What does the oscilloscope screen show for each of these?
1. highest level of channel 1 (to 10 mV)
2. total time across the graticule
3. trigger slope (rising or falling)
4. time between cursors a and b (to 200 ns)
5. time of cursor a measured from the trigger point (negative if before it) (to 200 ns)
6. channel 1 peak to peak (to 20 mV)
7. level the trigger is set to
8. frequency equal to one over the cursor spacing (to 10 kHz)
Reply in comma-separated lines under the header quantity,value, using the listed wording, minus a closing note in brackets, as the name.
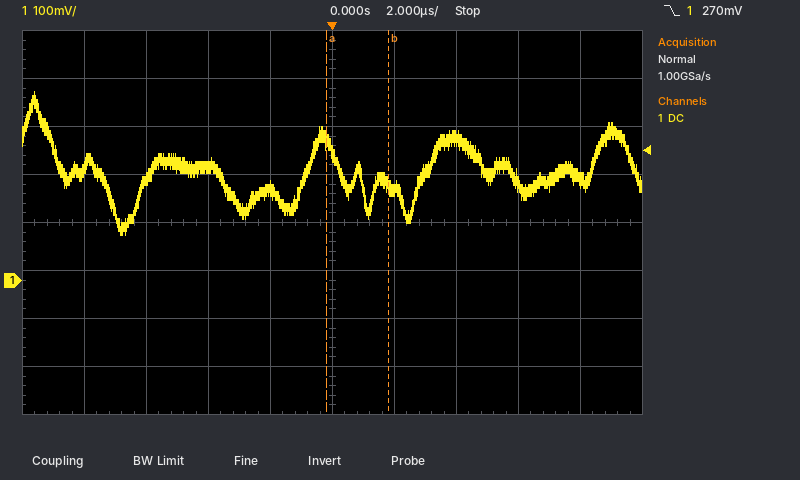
quantity,value
highest level of channel 1,390 mV
total time across the graticule,20 µs
trigger slope,falling
time between cursors a and b,2.0 µs
time of cursor a measured from the trigger point (negative if before it),-200 ns
channel 1 peak to peak,300 mV
level the trigger is set to,270 mV
frequency equal to one over the cursor spacing,500 kHz
